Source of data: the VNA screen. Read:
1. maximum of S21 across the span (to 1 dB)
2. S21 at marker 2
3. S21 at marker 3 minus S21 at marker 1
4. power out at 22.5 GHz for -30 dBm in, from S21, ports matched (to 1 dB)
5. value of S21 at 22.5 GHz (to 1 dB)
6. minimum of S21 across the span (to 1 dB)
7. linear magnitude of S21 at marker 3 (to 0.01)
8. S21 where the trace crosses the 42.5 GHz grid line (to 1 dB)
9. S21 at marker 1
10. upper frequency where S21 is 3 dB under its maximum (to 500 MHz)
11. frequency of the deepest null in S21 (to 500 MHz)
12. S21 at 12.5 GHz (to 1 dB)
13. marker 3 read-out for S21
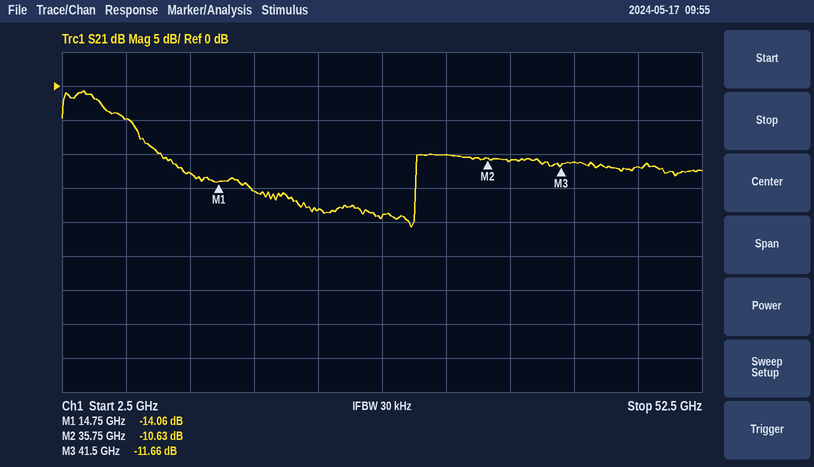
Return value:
-1 dB
-10.63 dB
2.40 dB
-48 dBm
-18 dB
-21 dB
0.26
-11 dB
-14.06 dB
6.0 GHz
30.0 GHz
-13 dB
-11.66 dB
